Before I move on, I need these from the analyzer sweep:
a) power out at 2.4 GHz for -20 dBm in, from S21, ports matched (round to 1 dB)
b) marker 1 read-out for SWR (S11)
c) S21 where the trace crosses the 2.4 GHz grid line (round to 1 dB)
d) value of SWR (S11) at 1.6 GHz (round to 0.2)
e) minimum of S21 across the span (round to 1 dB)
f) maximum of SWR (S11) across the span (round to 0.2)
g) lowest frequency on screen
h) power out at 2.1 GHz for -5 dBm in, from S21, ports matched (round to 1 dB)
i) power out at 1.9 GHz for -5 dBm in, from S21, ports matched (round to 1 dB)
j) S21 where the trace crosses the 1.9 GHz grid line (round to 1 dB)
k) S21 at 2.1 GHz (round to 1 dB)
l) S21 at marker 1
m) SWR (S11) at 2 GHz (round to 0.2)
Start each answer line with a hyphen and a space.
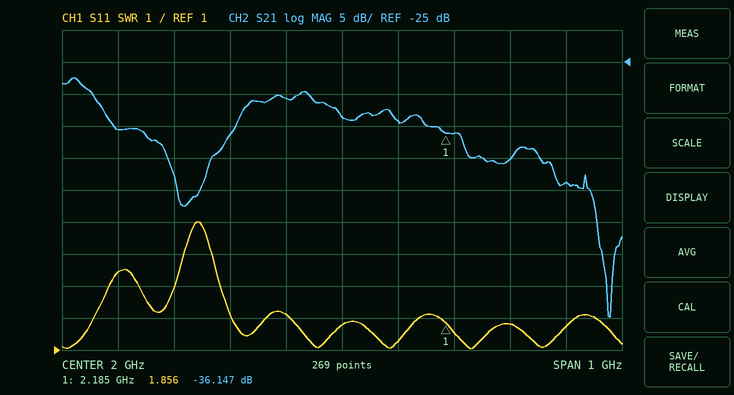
- -64 dBm
- 1.856
- -44 dB
- 3.4
- -65 dB
- 5.0
- 1.5 GHz
- -39 dBm
- -36 dBm
- -31 dB
- -34 dB
- -36.147 dB
- 1.8
